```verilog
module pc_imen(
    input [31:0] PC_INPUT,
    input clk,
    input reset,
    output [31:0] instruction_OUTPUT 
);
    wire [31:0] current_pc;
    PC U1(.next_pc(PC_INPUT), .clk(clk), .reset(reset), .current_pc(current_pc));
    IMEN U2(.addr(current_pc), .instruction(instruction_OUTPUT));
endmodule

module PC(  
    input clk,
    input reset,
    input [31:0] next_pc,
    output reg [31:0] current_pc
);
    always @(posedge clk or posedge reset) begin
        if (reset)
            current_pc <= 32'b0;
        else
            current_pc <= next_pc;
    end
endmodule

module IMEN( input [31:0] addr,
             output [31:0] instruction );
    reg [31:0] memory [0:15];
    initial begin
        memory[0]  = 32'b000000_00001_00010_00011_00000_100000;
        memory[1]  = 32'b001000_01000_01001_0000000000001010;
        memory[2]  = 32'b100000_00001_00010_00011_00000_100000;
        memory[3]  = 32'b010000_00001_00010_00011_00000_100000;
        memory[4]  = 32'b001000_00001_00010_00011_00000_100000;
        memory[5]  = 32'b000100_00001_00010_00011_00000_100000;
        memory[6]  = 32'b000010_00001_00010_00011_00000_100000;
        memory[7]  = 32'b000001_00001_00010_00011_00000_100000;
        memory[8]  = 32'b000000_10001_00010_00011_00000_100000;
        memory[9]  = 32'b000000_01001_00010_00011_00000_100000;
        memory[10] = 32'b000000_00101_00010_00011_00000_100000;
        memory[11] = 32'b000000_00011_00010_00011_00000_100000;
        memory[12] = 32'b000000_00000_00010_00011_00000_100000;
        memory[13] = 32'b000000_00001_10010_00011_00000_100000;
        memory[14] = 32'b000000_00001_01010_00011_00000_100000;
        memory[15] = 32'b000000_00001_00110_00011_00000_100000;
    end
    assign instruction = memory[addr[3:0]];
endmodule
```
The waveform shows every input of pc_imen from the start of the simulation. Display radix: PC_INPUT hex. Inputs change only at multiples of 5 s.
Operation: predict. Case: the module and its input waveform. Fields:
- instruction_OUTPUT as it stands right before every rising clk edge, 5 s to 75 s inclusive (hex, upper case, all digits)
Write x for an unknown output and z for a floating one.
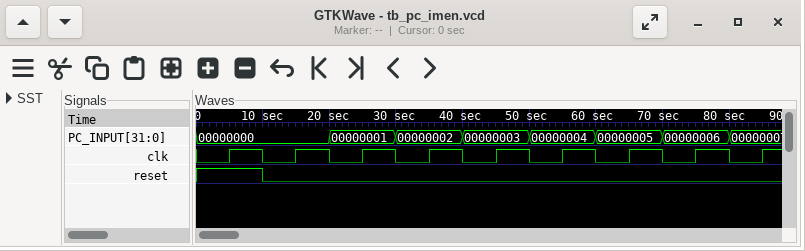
00221820, 00221820, 00221820, 2109000A, 80221820, 40221820, 20221820, 10221820
